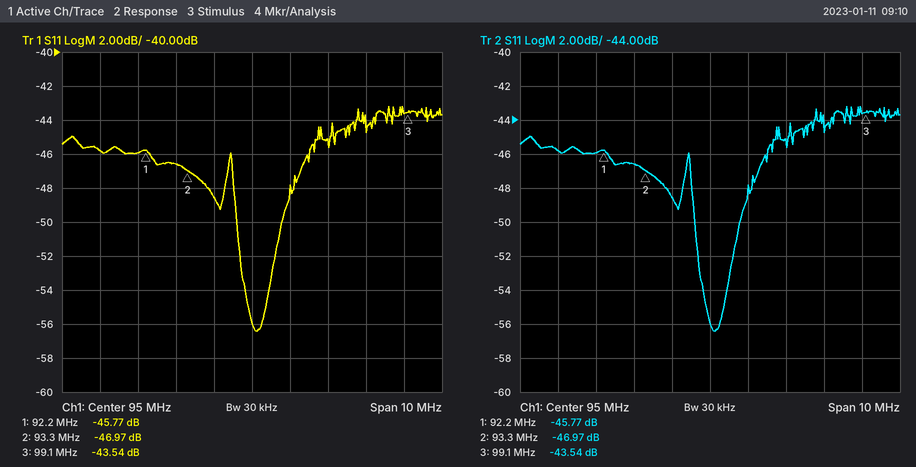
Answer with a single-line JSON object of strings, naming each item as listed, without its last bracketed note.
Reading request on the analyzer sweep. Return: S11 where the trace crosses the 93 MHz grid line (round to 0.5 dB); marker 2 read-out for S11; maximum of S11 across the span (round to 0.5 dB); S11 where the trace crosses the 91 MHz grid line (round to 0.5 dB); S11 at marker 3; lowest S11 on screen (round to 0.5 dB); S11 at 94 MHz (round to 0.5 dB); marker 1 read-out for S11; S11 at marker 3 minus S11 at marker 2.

{"S11 where the trace crosses the 93 MHz grid line": "-46.5 dB", "marker 2 read-out for S11": "-46.97 dB", "maximum of S11 across the span": "-43.0 dB", "S11 where the trace crosses the 91 MHz grid line": "-46.0 dB", "S11 at marker 3": "-43.54 dB", "lowest S11 on screen": "-56.5 dB", "S11 at 94 MHz": "-48.5 dB", "marker 1 read-out for S11": "-45.77 dB", "S11 at marker 3 minus S11 at marker 2": "3.43 dB"}
